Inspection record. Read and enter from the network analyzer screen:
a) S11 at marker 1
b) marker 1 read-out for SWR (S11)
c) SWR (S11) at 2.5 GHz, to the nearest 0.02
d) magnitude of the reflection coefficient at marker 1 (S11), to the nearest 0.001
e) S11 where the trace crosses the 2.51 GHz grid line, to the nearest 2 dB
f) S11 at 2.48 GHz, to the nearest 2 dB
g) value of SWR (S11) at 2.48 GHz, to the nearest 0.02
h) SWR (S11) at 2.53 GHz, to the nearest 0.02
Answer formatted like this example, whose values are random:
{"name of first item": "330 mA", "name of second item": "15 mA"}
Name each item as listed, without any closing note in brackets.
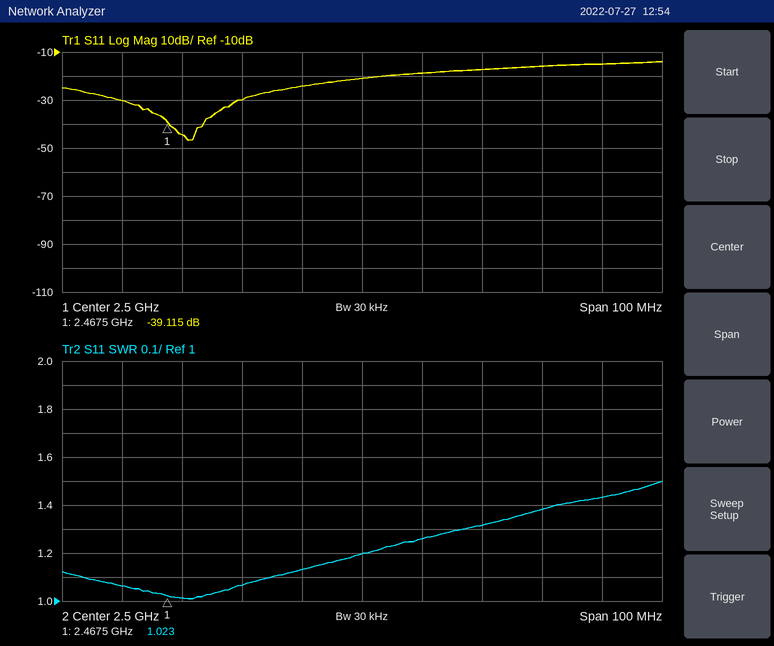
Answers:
{"S11 at marker 1": "-39.115 dB", "marker 1 read-out for SWR": "1.023", "SWR (S11) at 2.5 GHz, to the nearest 0.02": "1.20", "magnitude of the reflection coefficient at marker 1 (S11), to the nearest 0.001": "0.011", "S11 where the trace crosses the 2.51 GHz grid line, to the nearest 2 dB": "-18 dB", "S11 at 2.48 GHz, to the nearest 2 dB": "-30 dB", "value of SWR (S11) at 2.48 GHz, to the nearest 0.02": "1.06", "SWR (S11) at 2.53 GHz, to the nearest 0.02": "1.38"}
